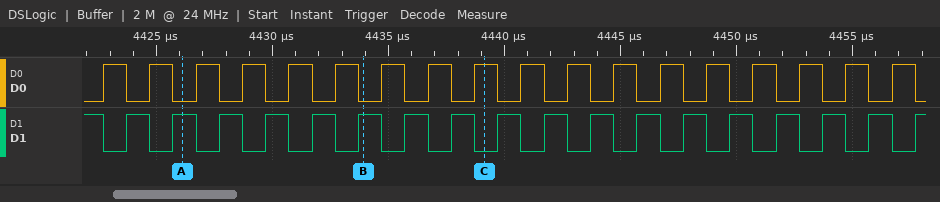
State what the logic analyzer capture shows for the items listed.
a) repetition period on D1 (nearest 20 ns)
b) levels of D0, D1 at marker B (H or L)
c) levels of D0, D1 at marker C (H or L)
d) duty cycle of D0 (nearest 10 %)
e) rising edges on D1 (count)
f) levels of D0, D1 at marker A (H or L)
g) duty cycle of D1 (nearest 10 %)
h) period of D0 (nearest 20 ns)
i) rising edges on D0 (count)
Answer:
2000 ns
D0=L, D1=H
D0=H, D1=L
50 %
18
D0=L, D1=H
50 %
2000 ns
18
